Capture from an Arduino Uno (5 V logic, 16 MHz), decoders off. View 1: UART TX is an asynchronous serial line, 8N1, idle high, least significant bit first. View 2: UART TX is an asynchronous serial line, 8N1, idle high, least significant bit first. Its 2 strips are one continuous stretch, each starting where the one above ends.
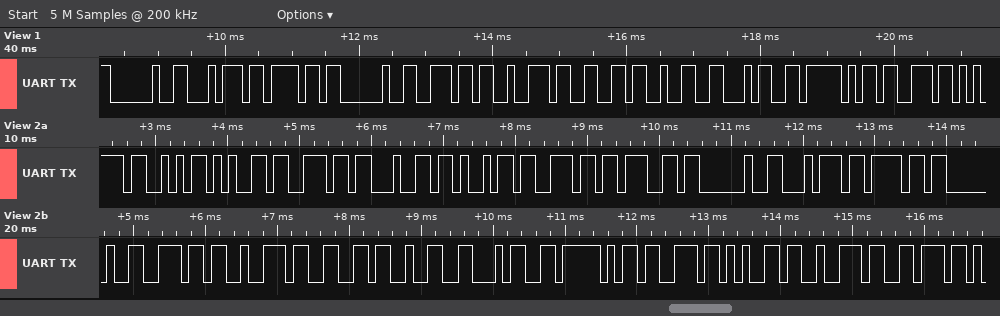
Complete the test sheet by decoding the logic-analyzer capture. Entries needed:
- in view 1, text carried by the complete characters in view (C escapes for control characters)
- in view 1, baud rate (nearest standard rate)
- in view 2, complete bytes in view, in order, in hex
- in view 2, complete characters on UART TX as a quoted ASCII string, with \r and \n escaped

" to nrf24_s"
9600 baud
53 65 6E 64 69 6E 67 20 74 6F 20 6E 72 66 32 34 5F 73 65 72 76
"Sending to nrf24_serv"
